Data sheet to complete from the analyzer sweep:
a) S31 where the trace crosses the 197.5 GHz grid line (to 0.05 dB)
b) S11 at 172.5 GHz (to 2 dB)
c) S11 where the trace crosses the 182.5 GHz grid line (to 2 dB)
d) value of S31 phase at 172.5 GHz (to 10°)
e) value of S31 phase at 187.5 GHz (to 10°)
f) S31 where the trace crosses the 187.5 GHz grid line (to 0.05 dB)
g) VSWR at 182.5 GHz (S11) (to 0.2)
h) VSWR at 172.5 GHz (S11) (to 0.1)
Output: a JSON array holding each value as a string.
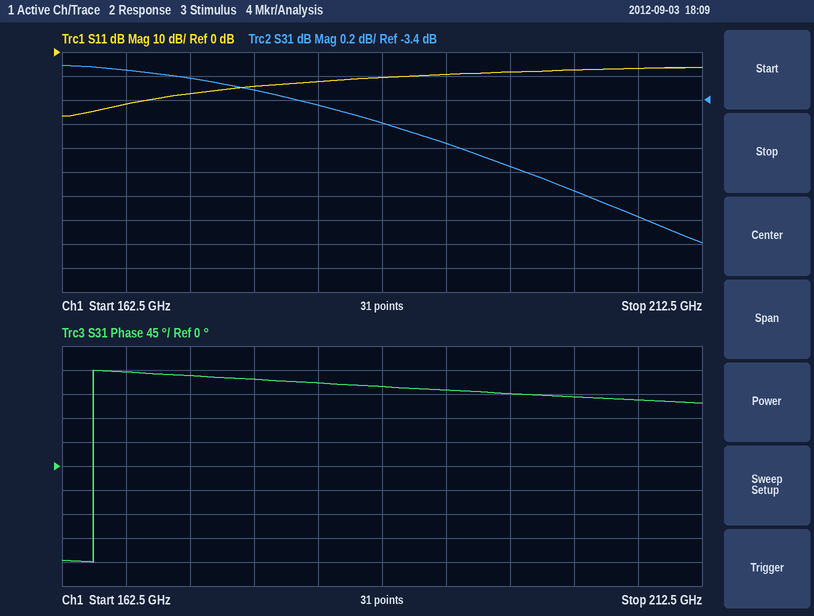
["-3.95 dB", "-18 dB", "-12 dB", "170°", "150°", "-3.60 dB", "1.6", "1.3"]
